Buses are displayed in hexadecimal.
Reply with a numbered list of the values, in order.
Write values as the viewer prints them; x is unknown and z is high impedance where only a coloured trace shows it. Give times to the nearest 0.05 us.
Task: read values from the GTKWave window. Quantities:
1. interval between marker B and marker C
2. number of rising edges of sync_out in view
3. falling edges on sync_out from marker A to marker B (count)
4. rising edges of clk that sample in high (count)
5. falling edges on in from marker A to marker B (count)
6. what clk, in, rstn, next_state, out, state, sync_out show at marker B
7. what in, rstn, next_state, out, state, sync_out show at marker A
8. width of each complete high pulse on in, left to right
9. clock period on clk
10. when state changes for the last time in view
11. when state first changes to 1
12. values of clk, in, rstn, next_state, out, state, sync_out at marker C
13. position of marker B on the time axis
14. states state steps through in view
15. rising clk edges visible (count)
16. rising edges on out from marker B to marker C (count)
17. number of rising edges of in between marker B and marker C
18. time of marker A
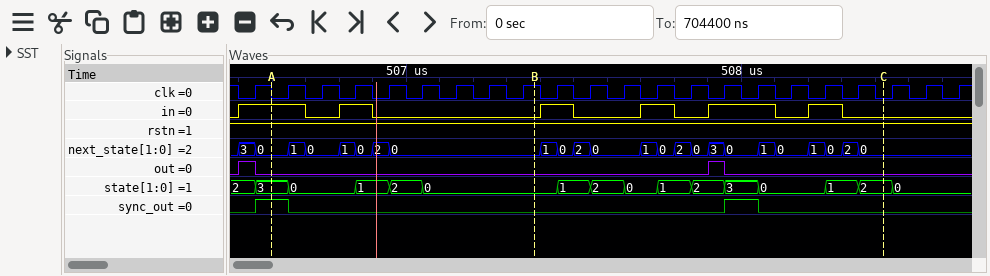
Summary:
1. 1.05 us
2. 2
3. 1
4. 8
5. 2
6. clk=1, in=0, rstn=1, next_state=0, out=0, state=0, sync_out=0
7. in=1, rstn=1, next_state=0, out=0, state=3, sync_out=1
8. 0.2 us, 0.1 us, 0.1 us, 0.1 us, 0.2 us, 0.1 us
9. 0.1 us
10. 508.45 us
11. 506.85 us
12. clk=0, in=0, rstn=1, next_state=0, out=0, state=2, sync_out=0
13. 507.4 us
14. 2, 3, 0, 1, 2, 0, 1, 2, 0, 1, 2, 3, 0, 1, 2, 0
15. 22
16. 1
17. 4
18. 506.6 us
